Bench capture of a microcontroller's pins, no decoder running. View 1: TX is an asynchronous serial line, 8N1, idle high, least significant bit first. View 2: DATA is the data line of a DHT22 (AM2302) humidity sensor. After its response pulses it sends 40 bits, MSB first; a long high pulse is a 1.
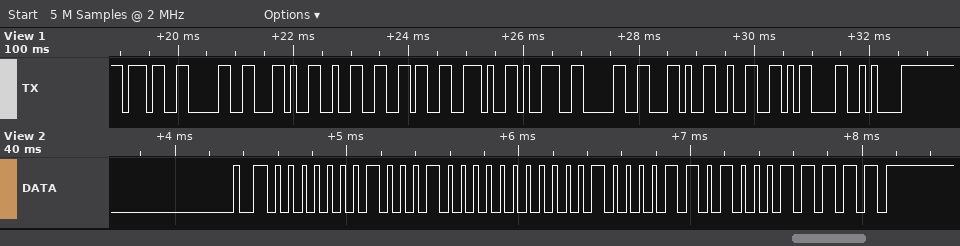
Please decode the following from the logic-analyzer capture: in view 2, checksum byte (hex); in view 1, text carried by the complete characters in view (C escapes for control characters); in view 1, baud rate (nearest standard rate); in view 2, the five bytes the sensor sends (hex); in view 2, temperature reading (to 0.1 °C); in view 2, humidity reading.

0x1F
"70,26.90,2\r\n"
9600 baud
01 10 01 0D 1F
26.9 °C
27.2 %
